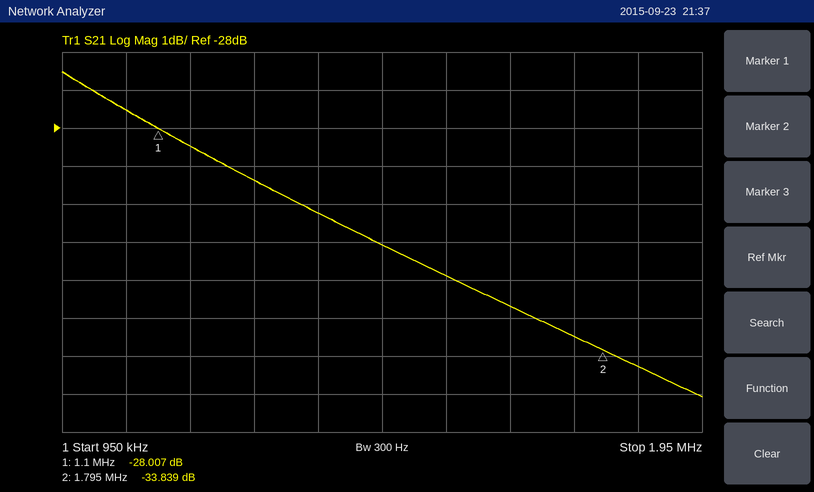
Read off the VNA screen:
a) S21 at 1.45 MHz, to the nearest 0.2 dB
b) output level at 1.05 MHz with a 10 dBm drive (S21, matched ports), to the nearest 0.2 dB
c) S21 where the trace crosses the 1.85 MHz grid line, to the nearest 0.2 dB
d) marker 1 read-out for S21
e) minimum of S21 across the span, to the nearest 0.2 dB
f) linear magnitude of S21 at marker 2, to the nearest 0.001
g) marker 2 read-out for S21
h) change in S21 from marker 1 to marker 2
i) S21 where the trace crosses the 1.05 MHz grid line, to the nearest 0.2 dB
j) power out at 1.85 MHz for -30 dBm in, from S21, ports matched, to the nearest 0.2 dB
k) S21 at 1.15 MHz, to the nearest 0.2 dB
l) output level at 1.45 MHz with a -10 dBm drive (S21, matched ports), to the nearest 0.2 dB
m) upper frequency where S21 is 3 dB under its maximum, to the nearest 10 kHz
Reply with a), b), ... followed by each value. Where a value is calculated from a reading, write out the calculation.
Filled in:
a) -31.0 dB
b) 10 dBm + (-27.6 dB) = -17.6 dBm
c) -34.2 dB
d) -28.007 dB
e) -35.0 dB
f) 10^(-33.839/20) ≈ 0.020
g) -33.839 dB
h) -33.839 − (-28.007) = -5.832 dB
i) -27.6 dB
j) -30 dBm + (-34.2 dB) = -64.2 dBm
k) -28.4 dB
l) -10 dBm + (-31.0 dB) = -41.0 dBm
m) 1.27 MHz
